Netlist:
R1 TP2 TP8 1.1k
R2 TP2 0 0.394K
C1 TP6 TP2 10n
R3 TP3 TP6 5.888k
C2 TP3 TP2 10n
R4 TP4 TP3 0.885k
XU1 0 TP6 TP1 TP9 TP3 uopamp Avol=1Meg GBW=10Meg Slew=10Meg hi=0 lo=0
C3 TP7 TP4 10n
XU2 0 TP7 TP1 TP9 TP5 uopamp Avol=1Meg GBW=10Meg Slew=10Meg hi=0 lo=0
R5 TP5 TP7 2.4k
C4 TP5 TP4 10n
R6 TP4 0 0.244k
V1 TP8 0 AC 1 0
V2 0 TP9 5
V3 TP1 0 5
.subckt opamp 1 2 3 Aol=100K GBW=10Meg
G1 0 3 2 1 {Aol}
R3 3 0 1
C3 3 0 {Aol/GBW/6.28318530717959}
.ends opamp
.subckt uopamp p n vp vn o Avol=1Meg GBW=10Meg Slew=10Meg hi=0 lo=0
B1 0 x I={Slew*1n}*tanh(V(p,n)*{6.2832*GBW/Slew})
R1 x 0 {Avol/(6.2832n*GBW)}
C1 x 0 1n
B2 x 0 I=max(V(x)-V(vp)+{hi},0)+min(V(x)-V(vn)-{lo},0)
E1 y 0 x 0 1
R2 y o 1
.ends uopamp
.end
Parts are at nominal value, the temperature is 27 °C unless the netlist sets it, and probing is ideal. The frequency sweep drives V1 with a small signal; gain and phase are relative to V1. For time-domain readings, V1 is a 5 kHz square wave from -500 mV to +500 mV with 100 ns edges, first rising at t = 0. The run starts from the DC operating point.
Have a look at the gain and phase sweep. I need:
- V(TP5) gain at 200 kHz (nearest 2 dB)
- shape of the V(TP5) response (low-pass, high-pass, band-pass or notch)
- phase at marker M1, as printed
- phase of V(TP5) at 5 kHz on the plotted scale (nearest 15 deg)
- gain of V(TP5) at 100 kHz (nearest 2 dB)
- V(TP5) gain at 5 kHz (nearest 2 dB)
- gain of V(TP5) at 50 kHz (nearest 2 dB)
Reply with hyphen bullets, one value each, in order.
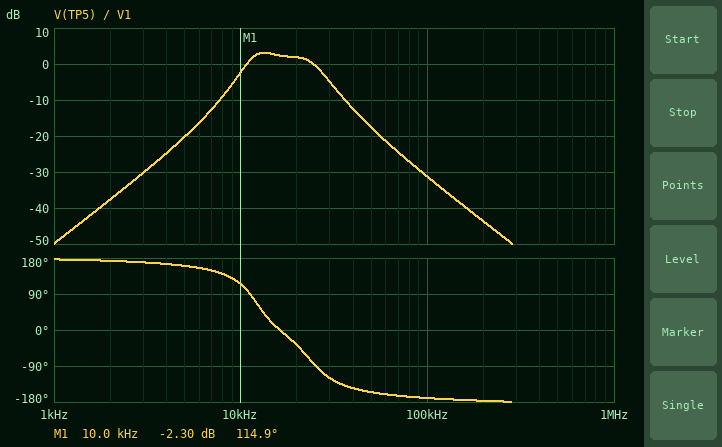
- -44 dB
- band-pass
- 114.9 deg
- 165 deg
- -32 dB
- -20 dB
- -18 dB
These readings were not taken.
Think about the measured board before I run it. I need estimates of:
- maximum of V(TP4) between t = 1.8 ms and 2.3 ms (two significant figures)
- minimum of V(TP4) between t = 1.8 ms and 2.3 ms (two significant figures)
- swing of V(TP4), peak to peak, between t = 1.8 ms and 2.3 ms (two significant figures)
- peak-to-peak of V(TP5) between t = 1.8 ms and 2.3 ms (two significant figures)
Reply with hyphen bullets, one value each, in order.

- 230 mV
- -230 mV
- 460 mV
- 830 mV
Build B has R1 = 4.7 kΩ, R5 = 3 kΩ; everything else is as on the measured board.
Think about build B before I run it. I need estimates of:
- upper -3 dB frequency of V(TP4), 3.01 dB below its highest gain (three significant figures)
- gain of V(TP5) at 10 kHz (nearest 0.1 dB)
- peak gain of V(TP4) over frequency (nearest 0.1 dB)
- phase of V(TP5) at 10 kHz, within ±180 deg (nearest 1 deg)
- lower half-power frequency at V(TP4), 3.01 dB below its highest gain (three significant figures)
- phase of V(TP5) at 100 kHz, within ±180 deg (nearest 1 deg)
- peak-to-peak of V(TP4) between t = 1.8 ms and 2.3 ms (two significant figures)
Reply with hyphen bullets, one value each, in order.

- 16.2 kHz
- -10.5 dB
- -15.1 dB
- 91 deg
- 8.90 kHz
- -172 deg
- 110 mV
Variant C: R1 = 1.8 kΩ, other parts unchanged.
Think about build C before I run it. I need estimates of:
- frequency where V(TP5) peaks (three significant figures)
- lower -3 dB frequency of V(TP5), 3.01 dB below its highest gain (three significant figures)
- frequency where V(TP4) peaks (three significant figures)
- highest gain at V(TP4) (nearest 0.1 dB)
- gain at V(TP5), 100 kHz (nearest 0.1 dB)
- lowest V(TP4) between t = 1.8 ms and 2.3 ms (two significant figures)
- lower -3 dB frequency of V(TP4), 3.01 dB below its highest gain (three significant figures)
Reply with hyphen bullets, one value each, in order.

- 12.7 kHz
- 10.2 kHz
- 11.8 kHz
- -7.1 dB
- -35.6 dB
- -140 mV
- 9.46 kHz
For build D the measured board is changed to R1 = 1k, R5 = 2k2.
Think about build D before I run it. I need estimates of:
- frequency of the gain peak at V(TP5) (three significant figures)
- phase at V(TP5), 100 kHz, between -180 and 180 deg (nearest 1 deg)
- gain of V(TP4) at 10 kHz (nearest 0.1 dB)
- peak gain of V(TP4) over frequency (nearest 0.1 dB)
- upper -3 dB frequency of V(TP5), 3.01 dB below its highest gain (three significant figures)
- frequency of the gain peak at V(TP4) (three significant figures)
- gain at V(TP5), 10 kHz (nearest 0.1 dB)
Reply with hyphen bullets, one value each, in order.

- 13.4 kHz
- -169 deg
- -5.5 dB
- -2.0 dB
- 24.8 kHz
- 12.6 kHz
- -2.7 dB
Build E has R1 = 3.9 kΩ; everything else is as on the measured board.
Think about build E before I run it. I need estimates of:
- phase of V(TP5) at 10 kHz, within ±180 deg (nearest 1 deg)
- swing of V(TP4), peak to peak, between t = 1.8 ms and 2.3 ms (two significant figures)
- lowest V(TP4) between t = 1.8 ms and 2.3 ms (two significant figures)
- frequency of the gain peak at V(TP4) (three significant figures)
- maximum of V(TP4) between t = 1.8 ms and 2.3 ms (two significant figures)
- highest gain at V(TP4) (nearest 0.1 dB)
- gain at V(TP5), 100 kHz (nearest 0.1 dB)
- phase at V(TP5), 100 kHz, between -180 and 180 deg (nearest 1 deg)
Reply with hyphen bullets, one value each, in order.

- 94 deg
- 130 mV
- -64 mV
- 11.2 kHz
- 64 mV
- -14.0 dB
- -42.3 dB
- -170 deg
